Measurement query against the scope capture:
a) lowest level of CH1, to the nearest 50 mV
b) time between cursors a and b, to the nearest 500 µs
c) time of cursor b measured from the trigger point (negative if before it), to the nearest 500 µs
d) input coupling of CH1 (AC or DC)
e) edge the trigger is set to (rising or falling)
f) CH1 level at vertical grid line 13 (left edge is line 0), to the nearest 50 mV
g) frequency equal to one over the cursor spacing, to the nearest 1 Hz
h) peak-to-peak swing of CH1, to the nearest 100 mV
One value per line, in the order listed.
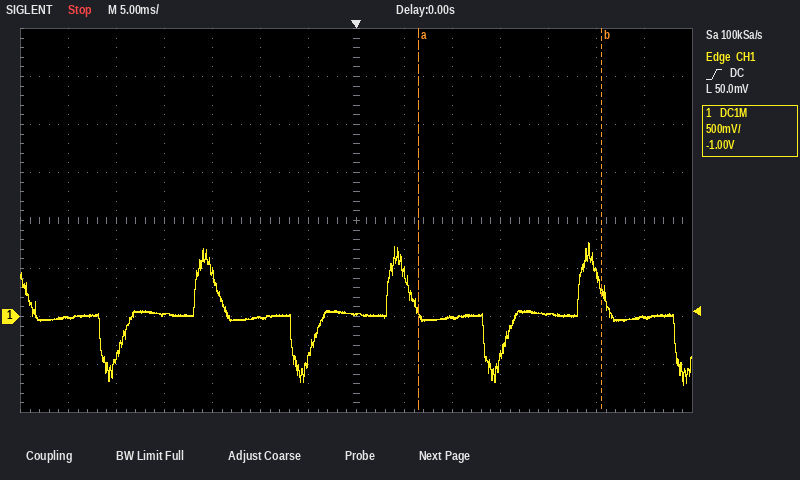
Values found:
-700 mV
19.0 ms
+25.5 ms
DC
rising
0 mV
53 Hz
1.50 V
